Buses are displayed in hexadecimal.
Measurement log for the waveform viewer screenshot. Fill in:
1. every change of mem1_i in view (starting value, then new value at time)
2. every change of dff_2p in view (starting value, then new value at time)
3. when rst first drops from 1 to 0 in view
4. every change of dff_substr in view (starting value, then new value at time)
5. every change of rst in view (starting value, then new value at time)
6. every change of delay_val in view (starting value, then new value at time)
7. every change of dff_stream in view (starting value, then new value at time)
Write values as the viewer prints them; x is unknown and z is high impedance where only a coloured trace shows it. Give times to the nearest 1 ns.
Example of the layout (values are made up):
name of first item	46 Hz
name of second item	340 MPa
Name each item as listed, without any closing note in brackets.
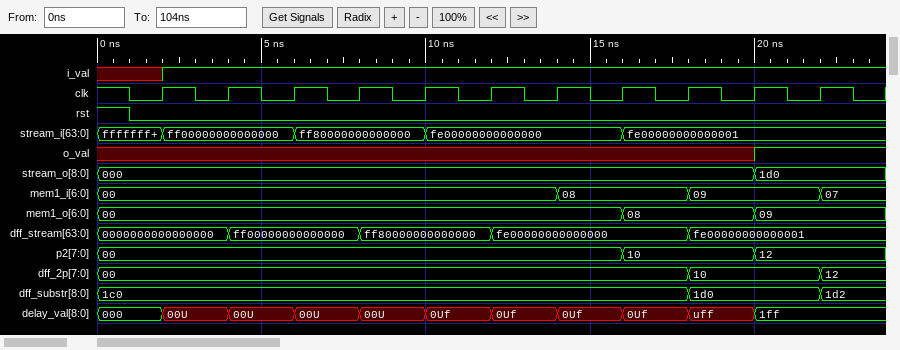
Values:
every change of mem1_i in view	00, 08 at 14 ns, 09 at 18 ns, 07 at 22 ns
every change of dff_2p in view	00, 10 at 18 ns, 12 at 22 ns
when rst first drops from 1 to 0 in view	1 ns
every change of dff_substr in view	1c0, 1d0 at 18 ns, 1d2 at 22 ns
every change of rst in view	1, 0 at 1 ns
every change of delay_val in view	000, 00U at 2 ns, 00U at 4 ns, 00U at 6 ns, 00U at 8 ns, 0Uf at 10 ns, 0Uf at 12 ns, 0Uf at 14 ns, 0Uf at 16 ns, uff at 18 ns, 1ff at 20 ns
every change of dff_stream in view	0000000000000000, ff00000000000000 at 4 ns, ff80000000000000 at 8 ns, fe00000000000000 at 12 ns, fe00000000000001 at 18 ns
